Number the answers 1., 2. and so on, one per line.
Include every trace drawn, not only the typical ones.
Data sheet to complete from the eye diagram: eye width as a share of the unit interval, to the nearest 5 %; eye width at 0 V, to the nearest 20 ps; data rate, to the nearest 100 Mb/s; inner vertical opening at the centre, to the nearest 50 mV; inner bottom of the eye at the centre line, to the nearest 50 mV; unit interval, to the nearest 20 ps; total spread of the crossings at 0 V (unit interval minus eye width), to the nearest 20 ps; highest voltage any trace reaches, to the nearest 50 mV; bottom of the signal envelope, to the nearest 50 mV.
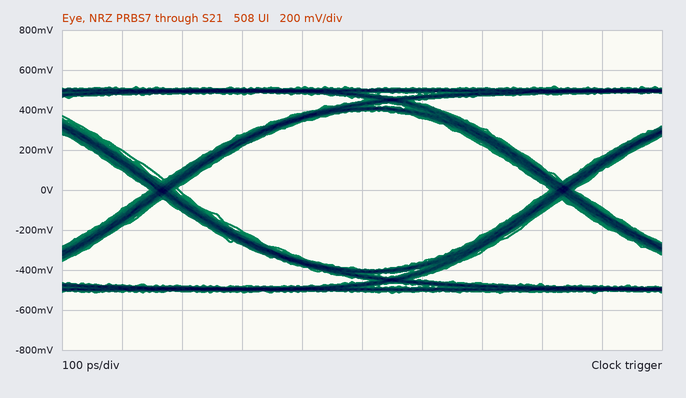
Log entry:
1. 95 %
2. 620 ps
3. 1.5 Gb/s
4. 800 mV
5. -400 mV
6. 660 ps
7. 40 ps
8. 500 mV
9. -500 mV
